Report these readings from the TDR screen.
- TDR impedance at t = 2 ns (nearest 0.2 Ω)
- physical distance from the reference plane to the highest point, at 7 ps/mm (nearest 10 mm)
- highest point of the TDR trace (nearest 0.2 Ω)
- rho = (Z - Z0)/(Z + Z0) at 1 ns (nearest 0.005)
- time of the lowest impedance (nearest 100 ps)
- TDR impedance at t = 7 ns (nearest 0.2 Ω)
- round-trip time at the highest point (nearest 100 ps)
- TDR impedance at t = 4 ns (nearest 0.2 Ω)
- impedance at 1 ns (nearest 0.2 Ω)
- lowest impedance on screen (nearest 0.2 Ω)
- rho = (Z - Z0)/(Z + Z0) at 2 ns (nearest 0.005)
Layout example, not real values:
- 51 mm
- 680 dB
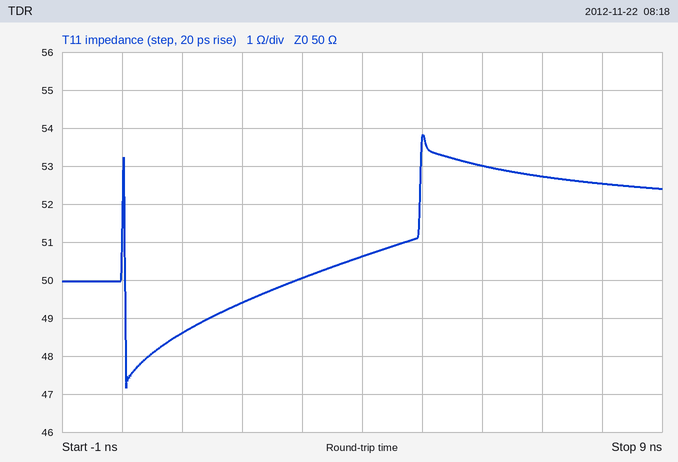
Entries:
- 49.4 Ω
- 360 mm
- 53.8 Ω
- -0.015
- 100 ps
- 52.8 Ω
- 5.0 ns
- 50.6 Ω
- 48.6 Ω
- 47.2 Ω
- -0.005
